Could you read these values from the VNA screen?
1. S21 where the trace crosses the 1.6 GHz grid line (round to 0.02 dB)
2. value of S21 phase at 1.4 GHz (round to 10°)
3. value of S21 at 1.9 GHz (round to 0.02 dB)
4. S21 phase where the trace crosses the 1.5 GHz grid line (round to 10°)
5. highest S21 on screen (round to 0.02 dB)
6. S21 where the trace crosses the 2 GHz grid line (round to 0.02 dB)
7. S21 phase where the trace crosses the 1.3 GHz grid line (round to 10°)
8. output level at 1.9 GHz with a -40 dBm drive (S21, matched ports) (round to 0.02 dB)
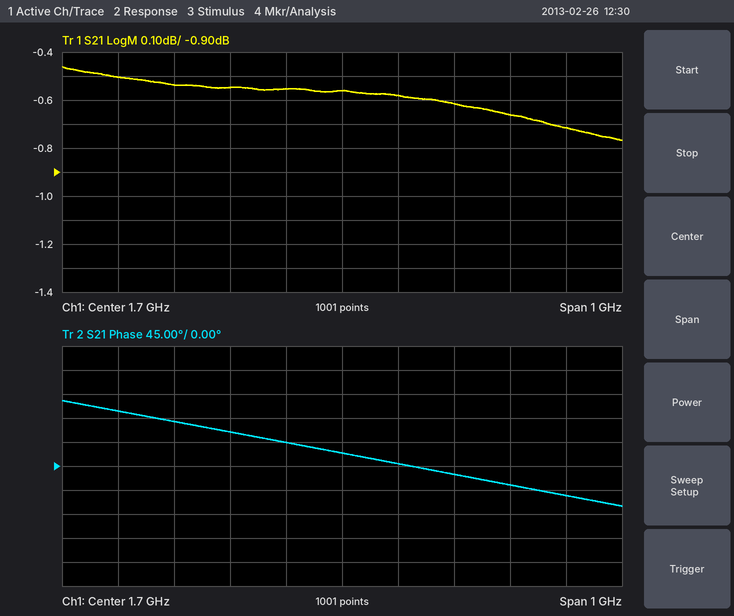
-0.56 dB
80°
-0.62 dB
60°
-0.46 dB
-0.66 dB
100°
-40.62 dBm
